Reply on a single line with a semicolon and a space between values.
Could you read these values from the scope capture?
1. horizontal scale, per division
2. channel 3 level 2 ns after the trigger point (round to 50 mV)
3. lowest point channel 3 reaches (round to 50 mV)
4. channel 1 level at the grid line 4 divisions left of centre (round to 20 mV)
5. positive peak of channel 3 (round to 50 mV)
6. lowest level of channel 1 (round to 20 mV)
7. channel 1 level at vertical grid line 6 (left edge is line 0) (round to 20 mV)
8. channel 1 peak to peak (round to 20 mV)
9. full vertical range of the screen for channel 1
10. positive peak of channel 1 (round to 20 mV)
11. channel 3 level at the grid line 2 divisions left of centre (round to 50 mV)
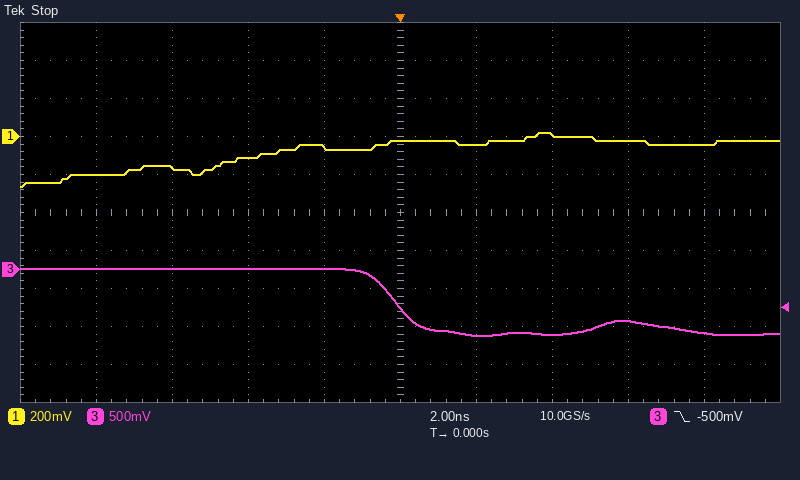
2 ns; -850 mV; -850 mV; -200 mV; 0 mV; -260 mV; -40 mV; 280 mV; 2 V; 20 mV; 0 mV
